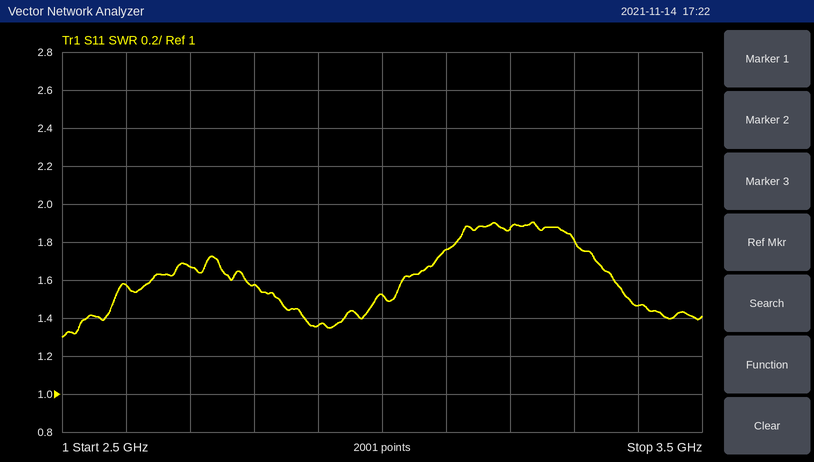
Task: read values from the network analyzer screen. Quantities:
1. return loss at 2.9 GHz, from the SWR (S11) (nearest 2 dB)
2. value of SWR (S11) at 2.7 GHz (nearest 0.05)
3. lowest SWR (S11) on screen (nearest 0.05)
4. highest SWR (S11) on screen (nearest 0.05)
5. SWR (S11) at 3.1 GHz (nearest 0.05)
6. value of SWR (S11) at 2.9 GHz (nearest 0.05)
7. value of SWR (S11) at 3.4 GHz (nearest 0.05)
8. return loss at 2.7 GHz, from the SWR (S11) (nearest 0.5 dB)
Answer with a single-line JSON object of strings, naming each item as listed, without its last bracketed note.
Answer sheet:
{"return loss at 2.9 GHz, from the SWR (S11)": "16 dB", "value of SWR (S11) at 2.7 GHz": "1.65", "lowest SWR (S11) on screen": "1.30", "highest SWR (S11) on screen": "1.90", "SWR (S11) at 3.1 GHz": "1.75", "value of SWR (S11) at 2.9 GHz": "1.35", "value of SWR (S11) at 3.4 GHz": "1.45", "return loss at 2.7 GHz, from the SWR (S11)": "12.0 dB"}
